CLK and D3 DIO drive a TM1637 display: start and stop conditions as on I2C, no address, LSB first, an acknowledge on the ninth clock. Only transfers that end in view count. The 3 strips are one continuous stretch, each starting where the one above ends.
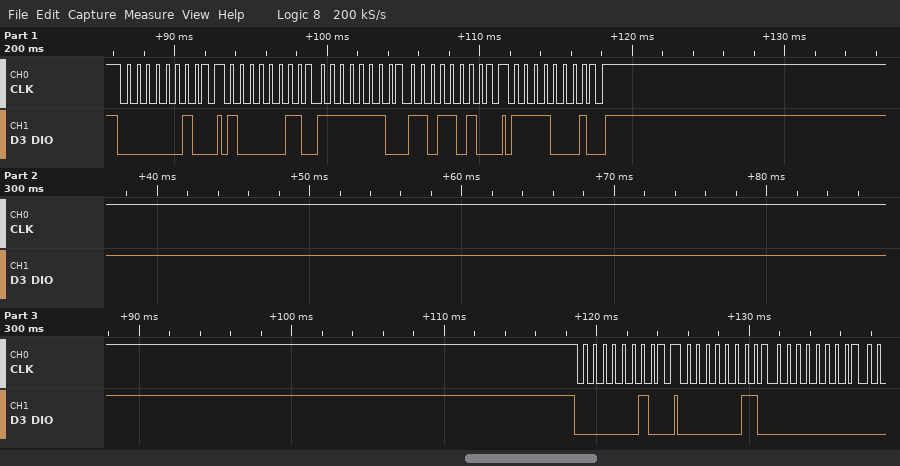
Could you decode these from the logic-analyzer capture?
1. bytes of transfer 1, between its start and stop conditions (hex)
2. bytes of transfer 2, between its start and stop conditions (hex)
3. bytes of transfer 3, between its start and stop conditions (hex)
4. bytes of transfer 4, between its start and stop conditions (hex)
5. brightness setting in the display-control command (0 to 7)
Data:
40
C1 7F 5B
8F
40
7
